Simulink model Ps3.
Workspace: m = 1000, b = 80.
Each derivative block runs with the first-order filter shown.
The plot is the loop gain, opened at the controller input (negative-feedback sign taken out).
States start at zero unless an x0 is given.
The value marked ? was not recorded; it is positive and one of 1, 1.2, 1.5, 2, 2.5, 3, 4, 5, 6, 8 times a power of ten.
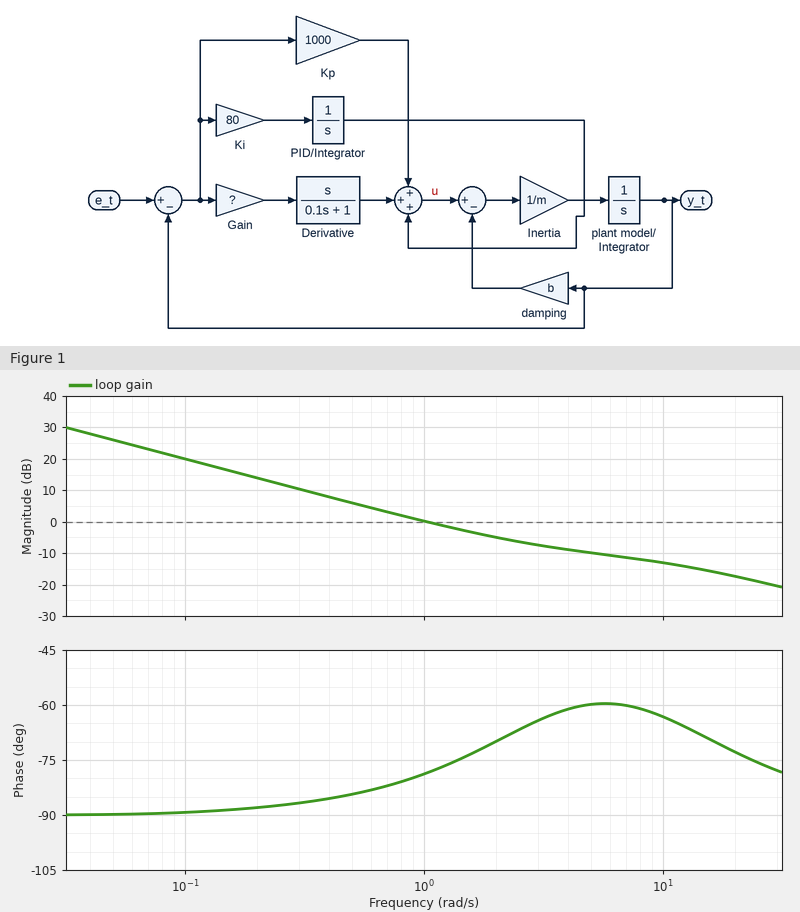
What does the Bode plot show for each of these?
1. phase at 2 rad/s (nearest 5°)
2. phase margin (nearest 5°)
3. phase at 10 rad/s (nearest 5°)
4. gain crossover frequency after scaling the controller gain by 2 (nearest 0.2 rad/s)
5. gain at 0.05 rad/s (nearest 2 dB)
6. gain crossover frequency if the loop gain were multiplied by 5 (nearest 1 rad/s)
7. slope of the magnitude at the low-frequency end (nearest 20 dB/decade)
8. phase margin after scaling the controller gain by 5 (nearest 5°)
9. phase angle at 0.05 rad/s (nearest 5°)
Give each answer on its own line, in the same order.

-70°
100°
-65°
2.4 rad/s
26 dB
12 rad/s
-20 dB/decade
115°
-90°
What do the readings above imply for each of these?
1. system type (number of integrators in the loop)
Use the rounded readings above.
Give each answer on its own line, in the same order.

1
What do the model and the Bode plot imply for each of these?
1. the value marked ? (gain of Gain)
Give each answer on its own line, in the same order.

200
